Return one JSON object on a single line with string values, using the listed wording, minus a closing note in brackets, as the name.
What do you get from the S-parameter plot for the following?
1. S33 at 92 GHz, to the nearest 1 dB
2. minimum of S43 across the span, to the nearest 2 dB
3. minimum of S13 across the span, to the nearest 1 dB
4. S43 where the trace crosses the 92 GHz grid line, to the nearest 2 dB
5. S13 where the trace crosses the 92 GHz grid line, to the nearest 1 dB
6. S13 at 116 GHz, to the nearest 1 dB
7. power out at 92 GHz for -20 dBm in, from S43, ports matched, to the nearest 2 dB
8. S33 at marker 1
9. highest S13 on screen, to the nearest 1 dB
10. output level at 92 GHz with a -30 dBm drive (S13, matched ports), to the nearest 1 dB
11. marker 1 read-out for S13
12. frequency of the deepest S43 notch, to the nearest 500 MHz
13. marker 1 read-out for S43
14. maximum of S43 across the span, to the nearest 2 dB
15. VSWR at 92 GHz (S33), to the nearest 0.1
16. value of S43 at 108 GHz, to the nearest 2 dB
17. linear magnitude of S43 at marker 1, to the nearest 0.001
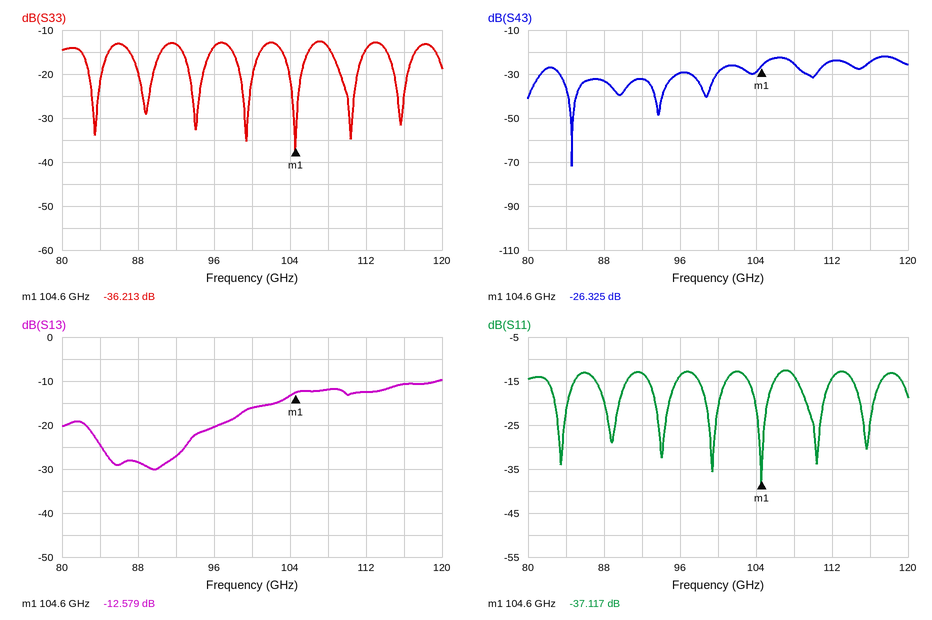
{"S33 at 92 GHz, to the nearest 1 dB": "-13 dB", "minimum of S43 across the span, to the nearest 2 dB": "-72 dB", "minimum of S13 across the span, to the nearest 1 dB": "-30 dB", "S43 where the trace crosses the 92 GHz grid line, to the nearest 2 dB": "-32 dB", "S13 where the trace crosses the 92 GHz grid line, to the nearest 1 dB": "-27 dB", "S13 at 116 GHz, to the nearest 1 dB": "-11 dB", "power out at 92 GHz for -20 dBm in, from S43, ports matched, to the nearest 2 dB": "-52 dBm", "S33 at marker 1": "-36.213 dB", "highest S13 on screen, to the nearest 1 dB": "-10 dB", "output level at 92 GHz with a -30 dBm drive (S13, matched ports), to the nearest 1 dB": "-57 dBm", "marker 1 read-out for S13": "-12.579 dB", "frequency of the deepest S43 notch, to the nearest 500 MHz": "84.5 GHz", "marker 1 read-out for S43": "-26.325 dB", "maximum of S43 across the span, to the nearest 2 dB": "-22 dB", "VSWR at 92 GHz (S33), to the nearest 0.1": "1.6", "value of S43 at 108 GHz, to the nearest 2 dB": "-26 dB", "linear magnitude of S43 at marker 1, to the nearest 0.001": "0.048"}
